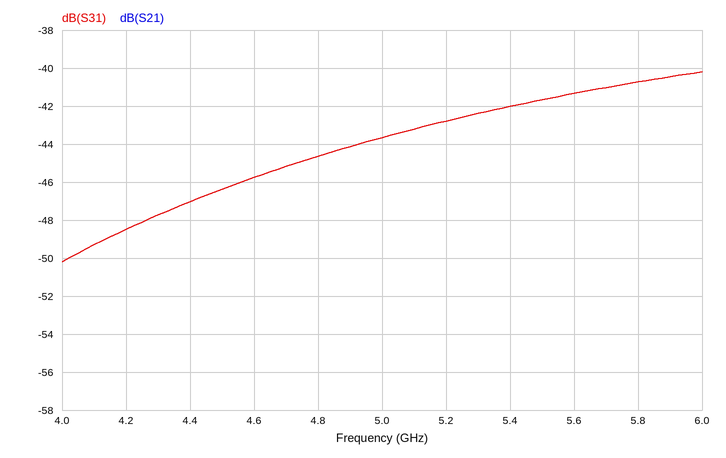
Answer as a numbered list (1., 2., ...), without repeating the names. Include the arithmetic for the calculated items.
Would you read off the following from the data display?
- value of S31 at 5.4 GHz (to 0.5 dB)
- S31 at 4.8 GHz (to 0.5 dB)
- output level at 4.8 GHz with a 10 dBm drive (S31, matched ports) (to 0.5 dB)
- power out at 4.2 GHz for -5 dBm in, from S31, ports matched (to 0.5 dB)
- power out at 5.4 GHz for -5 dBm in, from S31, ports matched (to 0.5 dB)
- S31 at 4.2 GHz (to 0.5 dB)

1. -42.0 dB
2. -44.5 dB
3. 10 dBm + (-44.5 dB) = -34.5 dBm
4. -5 dBm + (-48.5 dB) = -53.5 dBm
5. -5 dBm + (-42.0 dB) = -47.0 dBm
6. -48.5 dB
